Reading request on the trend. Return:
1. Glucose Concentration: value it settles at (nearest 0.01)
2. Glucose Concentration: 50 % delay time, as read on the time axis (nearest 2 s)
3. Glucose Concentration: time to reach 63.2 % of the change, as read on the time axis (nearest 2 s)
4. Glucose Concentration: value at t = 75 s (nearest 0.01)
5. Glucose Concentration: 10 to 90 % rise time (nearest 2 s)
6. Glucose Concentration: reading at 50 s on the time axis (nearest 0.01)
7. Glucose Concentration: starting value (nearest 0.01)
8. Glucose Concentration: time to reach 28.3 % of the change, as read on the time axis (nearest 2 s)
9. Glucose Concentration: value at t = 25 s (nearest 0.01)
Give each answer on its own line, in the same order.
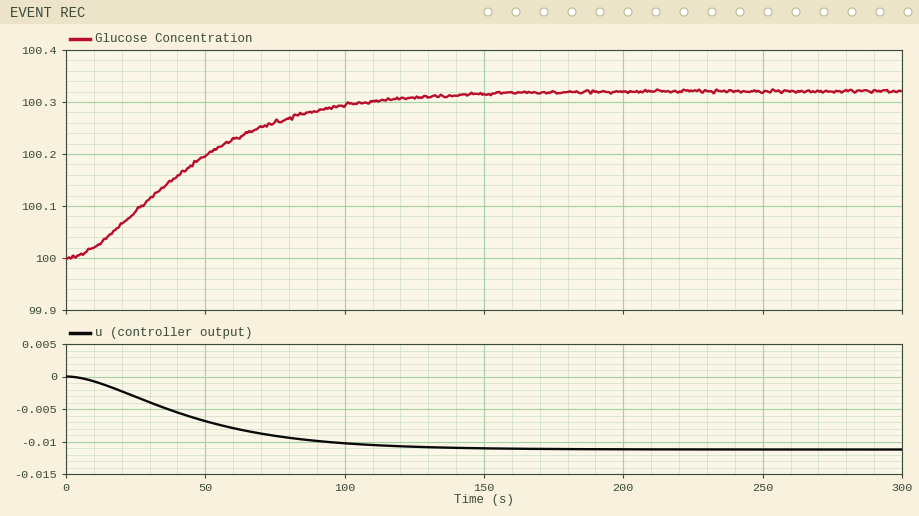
100.32
40 s
52 s
100.26
82 s
100.20
100.00
26 s
100.09
